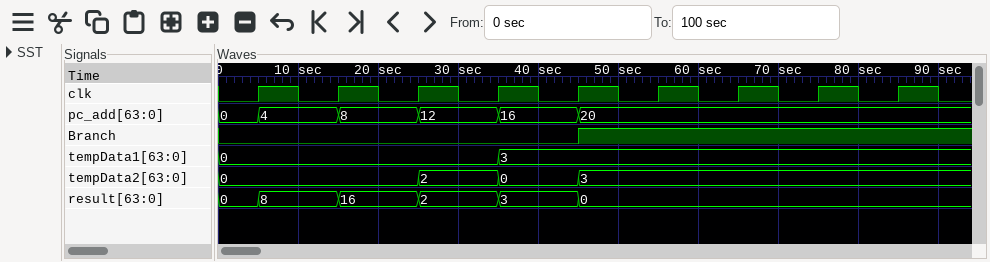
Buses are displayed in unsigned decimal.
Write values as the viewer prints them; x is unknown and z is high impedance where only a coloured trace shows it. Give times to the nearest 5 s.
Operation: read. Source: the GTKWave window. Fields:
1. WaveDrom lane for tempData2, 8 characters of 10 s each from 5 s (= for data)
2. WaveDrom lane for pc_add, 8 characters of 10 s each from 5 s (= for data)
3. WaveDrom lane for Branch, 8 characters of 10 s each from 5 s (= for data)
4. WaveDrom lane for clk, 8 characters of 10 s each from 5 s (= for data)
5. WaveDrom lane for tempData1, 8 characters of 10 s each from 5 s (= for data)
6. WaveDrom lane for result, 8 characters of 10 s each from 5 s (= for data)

{name: 'tempData2', wave: '=.===...', data: '0 2 0 3'}
{name: 'pc_add', wave: '=====...', data: '4 8 12 16 20'}
{name: 'Branch', wave: '0...1...'}
{name: 'clk', wave: 'p.......'}
{name: 'tempData1', wave: '=..=....', data: '0 3'}
{name: 'result', wave: '=====...', data: '8 16 2 3 0'}
